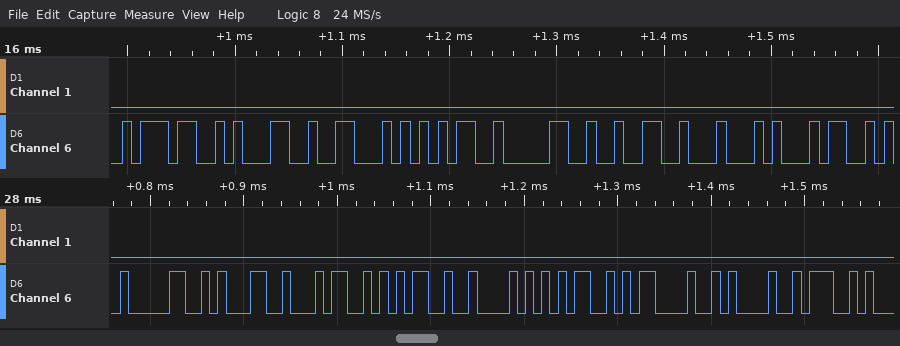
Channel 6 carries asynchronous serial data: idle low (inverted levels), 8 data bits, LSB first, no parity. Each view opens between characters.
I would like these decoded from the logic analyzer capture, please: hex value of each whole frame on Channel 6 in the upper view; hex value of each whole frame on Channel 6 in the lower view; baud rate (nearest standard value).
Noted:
91, 9D, 73, 95, 9F, 9B, 77, 97
9F, 9D, 97, 95, 7B, 95, E5, EB, 8B
115200 baud
